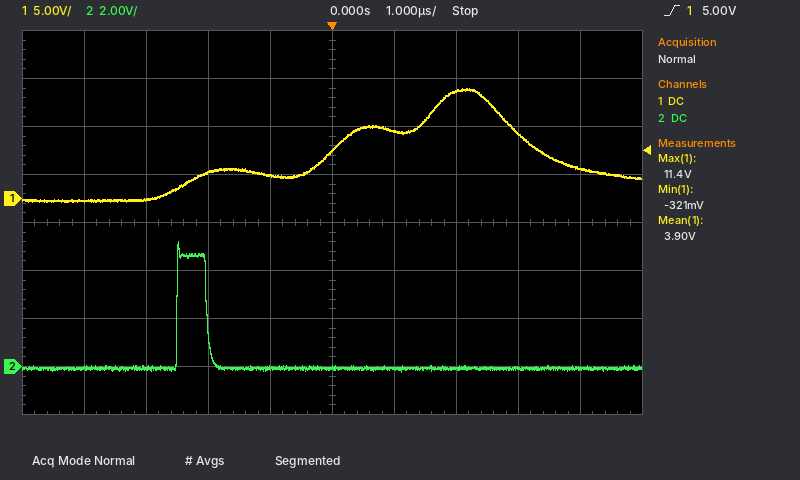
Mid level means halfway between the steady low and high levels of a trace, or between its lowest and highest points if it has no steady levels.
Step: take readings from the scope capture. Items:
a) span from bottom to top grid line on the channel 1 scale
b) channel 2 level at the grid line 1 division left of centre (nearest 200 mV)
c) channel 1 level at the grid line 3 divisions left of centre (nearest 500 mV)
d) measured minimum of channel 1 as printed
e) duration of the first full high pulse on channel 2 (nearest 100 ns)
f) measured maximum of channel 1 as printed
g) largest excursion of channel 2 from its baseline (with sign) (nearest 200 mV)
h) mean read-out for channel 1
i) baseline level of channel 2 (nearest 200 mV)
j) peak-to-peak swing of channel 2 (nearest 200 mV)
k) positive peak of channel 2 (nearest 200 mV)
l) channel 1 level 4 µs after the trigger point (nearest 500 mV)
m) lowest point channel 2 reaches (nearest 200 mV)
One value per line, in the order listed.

40 V
0.0 V
0.0 V
-321 mV
500 ns
11.4 V
+5.2 V
3.90 V
0.0 V
5.4 V
5.2 V
3.0 V
-200 mV
